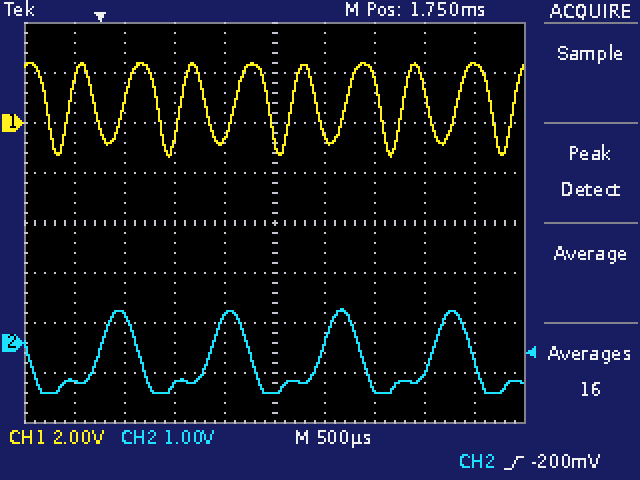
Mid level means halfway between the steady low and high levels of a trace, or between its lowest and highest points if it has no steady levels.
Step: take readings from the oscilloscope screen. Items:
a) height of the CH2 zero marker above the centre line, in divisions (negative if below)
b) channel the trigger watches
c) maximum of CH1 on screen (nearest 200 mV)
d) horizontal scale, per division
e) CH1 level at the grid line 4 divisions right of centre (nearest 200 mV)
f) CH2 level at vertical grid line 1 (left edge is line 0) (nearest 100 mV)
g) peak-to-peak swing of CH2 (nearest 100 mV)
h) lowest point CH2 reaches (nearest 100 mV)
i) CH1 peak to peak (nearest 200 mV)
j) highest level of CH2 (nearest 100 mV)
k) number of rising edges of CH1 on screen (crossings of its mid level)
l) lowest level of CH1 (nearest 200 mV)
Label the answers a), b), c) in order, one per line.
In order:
a) -2.4 div
b) CH2
c) 2.4 V
d) 500 µs
e) 2.4 V
f) -800 mV
g) 1.7 V
h) -1.0 V
i) 3.8 V
j) 700 mV
k) 9
l) -1.4 V
